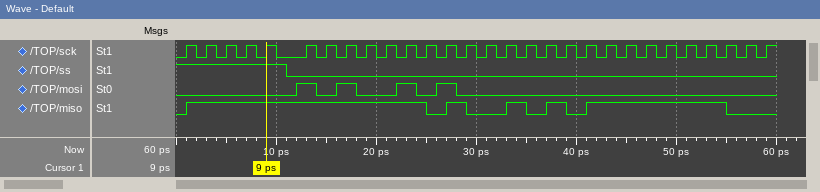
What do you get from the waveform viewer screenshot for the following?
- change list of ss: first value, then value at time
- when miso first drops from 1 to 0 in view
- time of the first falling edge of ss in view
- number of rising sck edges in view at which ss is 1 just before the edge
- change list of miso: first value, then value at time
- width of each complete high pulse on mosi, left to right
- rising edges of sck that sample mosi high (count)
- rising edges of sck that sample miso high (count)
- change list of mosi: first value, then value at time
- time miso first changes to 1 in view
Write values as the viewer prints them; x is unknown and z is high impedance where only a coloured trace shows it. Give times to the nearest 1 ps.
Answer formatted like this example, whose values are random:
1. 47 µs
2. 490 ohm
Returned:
1. 1, 0 at 11 ps
2. 25 ps
3. 11 ps
4. 5
5. 0, 1 at 1 ps, 0 at 25 ps, 1 at 27 ps, 0 at 29 ps, 1 at 33 ps, 0 at 35 ps, 1 at 37 ps, 0 at 39 ps, 1 at 41 ps, 0 at 55 ps
6. 2 ps, 2 ps, 2 ps, 2 ps
7. 4
8. 21
9. 0, 1 at 12 ps, 0 at 14 ps, 1 at 16 ps, 0 at 18 ps, 1 at 22 ps, 0 at 24 ps, 1 at 26 ps, 0 at 28 ps
10. 1 ps
